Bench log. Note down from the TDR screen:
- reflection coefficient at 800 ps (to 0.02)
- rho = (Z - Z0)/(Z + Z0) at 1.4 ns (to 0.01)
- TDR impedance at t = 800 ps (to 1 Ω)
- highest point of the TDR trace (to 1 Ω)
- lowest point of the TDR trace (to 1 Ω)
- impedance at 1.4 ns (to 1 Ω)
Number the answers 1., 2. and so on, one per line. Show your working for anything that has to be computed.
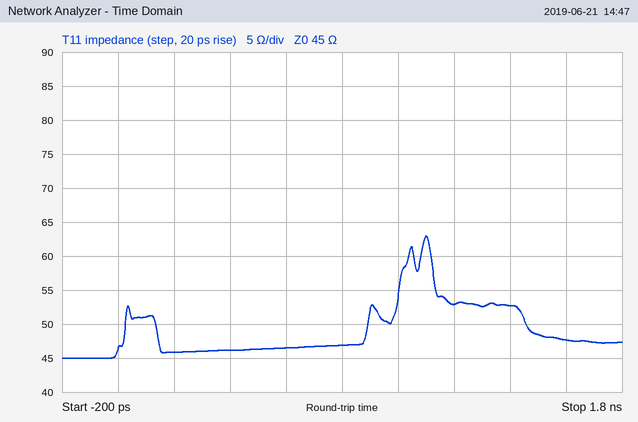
1. (47 − 45)/(47 + 45) ≈ +0.02
2. (53 − 45)/(53 + 45) ≈ +0.08
3. 47 Ω
4. 63 Ω
5. 45 Ω
6. 53 Ω
